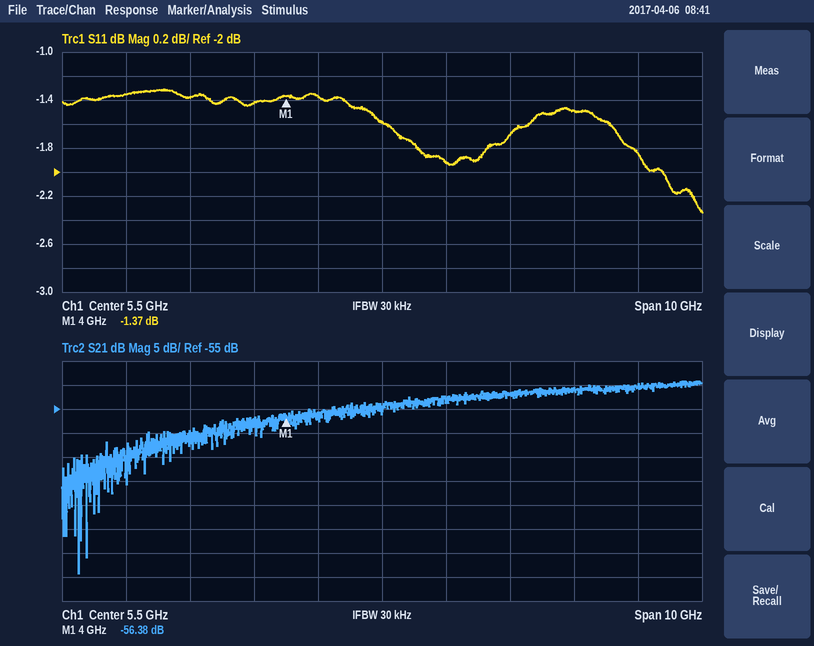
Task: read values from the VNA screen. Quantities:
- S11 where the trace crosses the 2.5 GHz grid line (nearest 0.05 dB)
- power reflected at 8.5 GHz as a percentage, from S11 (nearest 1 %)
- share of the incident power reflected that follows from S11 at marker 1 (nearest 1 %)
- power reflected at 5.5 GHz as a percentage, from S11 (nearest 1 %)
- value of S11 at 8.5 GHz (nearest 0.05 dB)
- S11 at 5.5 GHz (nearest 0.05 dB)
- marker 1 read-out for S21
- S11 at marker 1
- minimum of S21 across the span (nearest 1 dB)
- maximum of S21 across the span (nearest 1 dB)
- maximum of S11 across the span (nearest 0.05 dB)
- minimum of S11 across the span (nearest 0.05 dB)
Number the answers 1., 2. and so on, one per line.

1. -1.40 dB
2. 71 %
3. 73 %
4. 69 %
5. -1.50 dB
6. -1.60 dB
7. -56.38 dB
8. -1.37 dB
9. -89 dB
10. -49 dB
11. -1.30 dB
12. -2.35 dB
